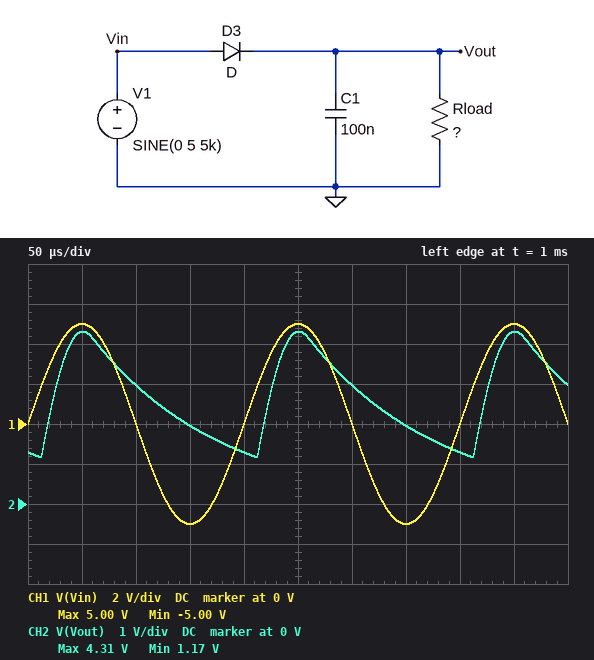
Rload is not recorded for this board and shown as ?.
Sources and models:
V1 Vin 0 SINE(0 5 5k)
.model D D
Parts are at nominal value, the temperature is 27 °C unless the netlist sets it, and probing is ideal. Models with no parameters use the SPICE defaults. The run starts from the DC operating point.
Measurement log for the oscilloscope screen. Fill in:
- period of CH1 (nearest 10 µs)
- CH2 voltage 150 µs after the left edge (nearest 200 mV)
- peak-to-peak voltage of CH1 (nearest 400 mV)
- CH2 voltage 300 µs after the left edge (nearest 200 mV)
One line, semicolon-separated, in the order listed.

200 µs; 2.0 V; 10.0 V; 3.0 V
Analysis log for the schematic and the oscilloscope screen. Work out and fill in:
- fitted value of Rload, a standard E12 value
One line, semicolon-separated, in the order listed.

1.2 kΩ
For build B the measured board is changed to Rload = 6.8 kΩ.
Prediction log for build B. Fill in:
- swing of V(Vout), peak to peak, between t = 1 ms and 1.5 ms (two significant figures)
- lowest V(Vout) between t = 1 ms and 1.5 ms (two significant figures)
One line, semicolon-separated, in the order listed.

990 mV; 3.4 V
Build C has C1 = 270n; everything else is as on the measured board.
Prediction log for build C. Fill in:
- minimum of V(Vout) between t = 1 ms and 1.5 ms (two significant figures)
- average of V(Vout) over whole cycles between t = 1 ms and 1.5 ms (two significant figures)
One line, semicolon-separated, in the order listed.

2.6 V; 3.4 V
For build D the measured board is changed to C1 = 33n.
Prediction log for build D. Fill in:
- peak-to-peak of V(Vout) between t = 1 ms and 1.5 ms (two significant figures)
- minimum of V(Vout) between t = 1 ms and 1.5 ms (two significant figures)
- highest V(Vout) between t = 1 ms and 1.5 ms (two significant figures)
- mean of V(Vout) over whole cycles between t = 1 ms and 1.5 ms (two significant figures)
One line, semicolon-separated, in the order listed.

4.2 V; 120 mV; 4.3 V; 1.7 V
